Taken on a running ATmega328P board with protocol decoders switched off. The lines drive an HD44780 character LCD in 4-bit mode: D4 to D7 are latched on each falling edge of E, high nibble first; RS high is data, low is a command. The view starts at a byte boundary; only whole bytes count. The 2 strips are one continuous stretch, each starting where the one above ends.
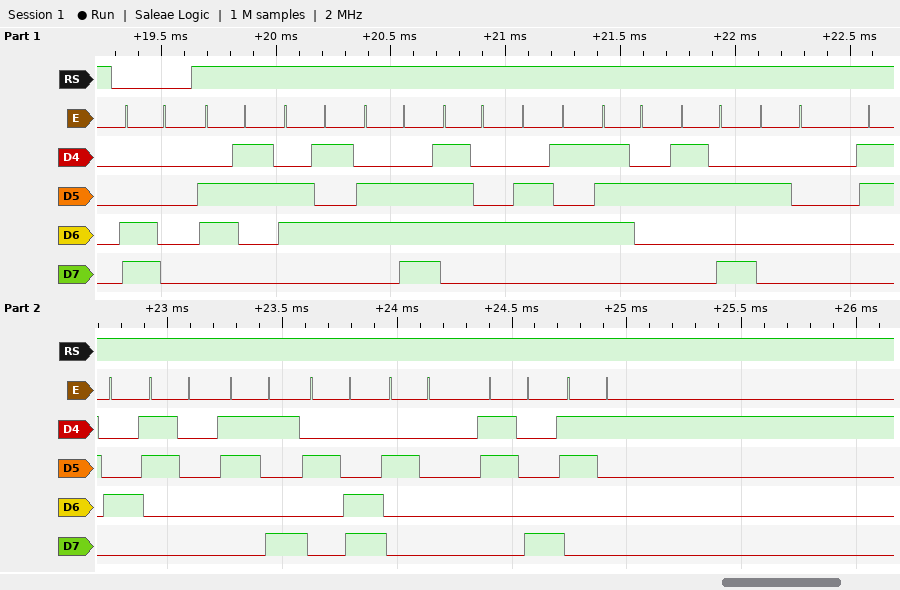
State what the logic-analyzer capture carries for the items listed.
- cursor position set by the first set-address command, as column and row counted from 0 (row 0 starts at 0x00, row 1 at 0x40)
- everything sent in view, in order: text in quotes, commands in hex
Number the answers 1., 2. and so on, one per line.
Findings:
1. column 0, row 1
2. 0xC0 "center: 409, 81"
